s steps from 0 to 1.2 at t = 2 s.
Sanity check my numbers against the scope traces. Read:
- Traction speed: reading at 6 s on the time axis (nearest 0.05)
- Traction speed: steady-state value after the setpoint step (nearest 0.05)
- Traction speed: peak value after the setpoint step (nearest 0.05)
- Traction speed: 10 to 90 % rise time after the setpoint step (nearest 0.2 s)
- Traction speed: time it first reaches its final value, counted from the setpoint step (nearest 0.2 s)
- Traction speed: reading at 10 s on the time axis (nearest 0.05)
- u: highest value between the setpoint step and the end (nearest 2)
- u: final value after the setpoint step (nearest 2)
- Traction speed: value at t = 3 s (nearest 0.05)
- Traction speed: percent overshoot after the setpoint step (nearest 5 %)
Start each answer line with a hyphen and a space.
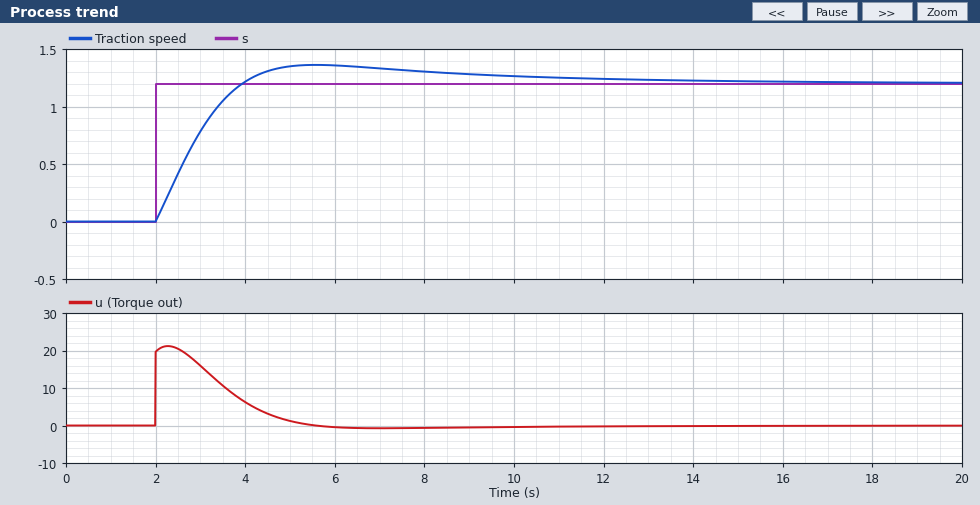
- 1.35
- 1.20
- 1.35
- 1.4 s
- 2.0 s
- 1.25
- 22
- 0
- 0.80
- 15 %
